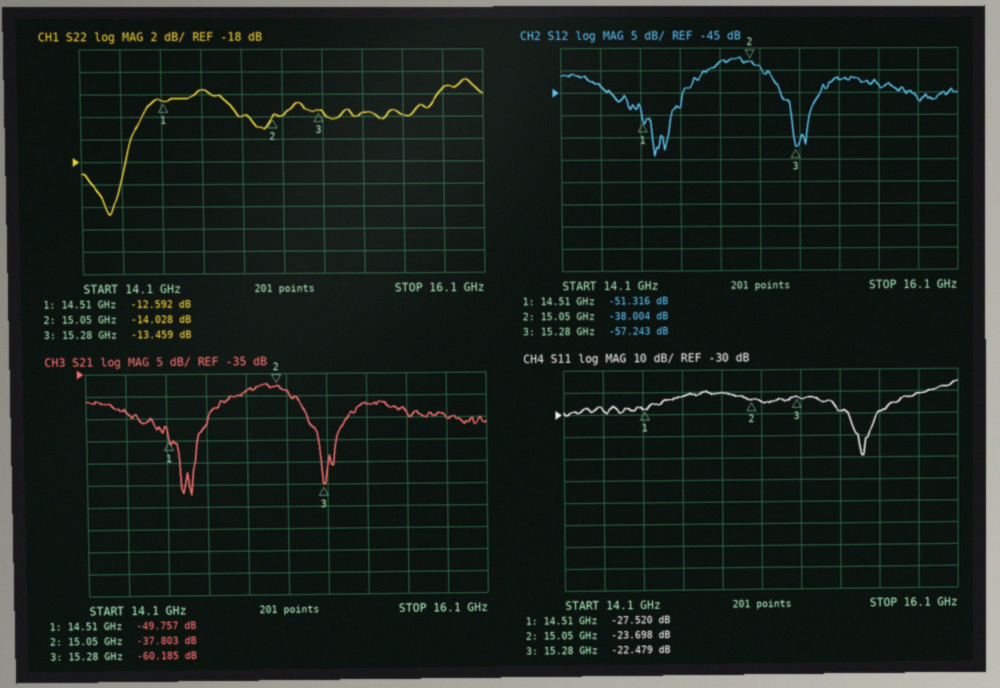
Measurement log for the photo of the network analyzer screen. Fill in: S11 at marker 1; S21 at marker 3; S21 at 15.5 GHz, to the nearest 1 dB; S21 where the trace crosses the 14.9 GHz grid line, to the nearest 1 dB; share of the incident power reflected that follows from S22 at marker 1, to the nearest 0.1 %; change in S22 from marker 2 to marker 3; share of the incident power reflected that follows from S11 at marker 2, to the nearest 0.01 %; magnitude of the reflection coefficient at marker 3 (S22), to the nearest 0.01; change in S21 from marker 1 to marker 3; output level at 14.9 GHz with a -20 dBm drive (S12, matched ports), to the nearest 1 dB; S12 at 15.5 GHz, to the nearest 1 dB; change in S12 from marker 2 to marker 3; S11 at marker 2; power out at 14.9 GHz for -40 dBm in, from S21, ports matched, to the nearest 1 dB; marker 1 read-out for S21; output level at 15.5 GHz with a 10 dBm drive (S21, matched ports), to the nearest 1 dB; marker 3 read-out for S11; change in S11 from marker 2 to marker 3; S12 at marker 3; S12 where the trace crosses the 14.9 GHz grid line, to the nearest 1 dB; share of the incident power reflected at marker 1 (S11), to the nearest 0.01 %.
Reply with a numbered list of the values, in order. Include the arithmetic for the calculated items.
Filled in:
1. -27.520 dB
2. -60.185 dB
3. -42 dB
4. -39 dB
5. 10^(-12.592/10) ≈ 5.5 %
6. -13.459 − (-14.028) = 0.569 dB
7. 10^(-23.698/10) ≈ 0.43 %
8. 10^(-13.459/20) ≈ 0.21
9. -60.185 − (-49.757) = -10.428 dB
10. -20 dBm + (-38 dB) = -58 dBm
11. -42 dB
12. -57.243 − (-38.004) = -19.239 dB
13. -23.698 dB
14. -40 dBm + (-39 dB) = -79 dBm
15. -49.757 dB
16. 10 dBm + (-42 dB) = -32 dBm
17. -22.479 dB
18. -22.479 − (-23.698) = 1.219 dB
19. -57.243 dB
20. -38 dB
21. 10^(-27.52/10) ≈ 0.18 %
